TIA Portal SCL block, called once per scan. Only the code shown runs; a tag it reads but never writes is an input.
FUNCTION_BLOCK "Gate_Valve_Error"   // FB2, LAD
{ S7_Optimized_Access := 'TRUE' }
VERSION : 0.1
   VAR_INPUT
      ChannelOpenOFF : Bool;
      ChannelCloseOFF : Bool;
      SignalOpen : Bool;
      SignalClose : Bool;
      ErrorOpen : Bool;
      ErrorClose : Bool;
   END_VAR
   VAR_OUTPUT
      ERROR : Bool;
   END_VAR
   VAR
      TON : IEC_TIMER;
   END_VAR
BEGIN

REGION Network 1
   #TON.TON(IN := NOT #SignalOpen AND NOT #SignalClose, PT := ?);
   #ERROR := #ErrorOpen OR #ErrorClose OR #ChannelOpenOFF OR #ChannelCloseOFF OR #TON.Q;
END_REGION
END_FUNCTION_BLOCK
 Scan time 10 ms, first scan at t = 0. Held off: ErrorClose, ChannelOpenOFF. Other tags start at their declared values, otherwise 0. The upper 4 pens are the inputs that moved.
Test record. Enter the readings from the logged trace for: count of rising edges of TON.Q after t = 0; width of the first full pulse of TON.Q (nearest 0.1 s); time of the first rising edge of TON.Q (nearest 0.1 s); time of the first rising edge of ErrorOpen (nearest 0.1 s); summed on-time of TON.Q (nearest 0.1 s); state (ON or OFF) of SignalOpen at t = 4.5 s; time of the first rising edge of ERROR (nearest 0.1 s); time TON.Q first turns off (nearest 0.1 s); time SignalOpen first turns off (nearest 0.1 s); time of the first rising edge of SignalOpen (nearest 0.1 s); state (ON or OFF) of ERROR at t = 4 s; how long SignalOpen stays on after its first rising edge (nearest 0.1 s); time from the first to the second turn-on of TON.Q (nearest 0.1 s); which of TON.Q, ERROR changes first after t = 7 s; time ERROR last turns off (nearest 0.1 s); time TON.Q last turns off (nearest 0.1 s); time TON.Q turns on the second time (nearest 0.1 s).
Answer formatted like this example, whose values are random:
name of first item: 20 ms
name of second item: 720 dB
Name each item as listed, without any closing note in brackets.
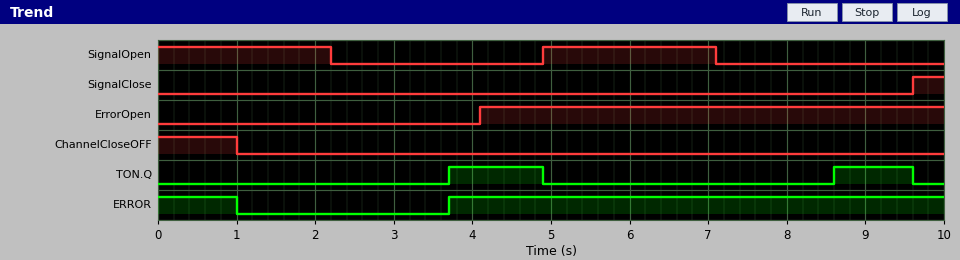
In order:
count of rising edges of TON.Q after t = 0: 2
width of the first full pulse of TON.Q: 1.2 s
time of the first rising edge of TON.Q: 3.7 s
time of the first rising edge of ErrorOpen: 4.1 s
summed on-time of TON.Q: 2.2 s
state (ON or OFF) of SignalOpen at t = 4.5 s: OFF
time of the first rising edge of ERROR: 3.7 s
time TON.Q first turns off: 4.9 s
time SignalOpen first turns off: 2.2 s
time of the first rising edge of SignalOpen: 4.9 s
state (ON or OFF) of ERROR at t = 4 s: ON
how long SignalOpen stays on after its first rising edge: 2.2 s
time from the first to the second turn-on of TON.Q: 4.9 s
which of TON.Q, ERROR changes first after t = 7 s: TON.Q
time ERROR last turns off: 1.0 s
time TON.Q last turns off: 9.6 s
time TON.Q turns on the second time: 8.6 s
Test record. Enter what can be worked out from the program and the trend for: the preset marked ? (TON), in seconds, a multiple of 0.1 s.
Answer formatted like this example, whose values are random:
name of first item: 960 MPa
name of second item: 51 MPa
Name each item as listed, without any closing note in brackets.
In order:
the preset marked ? (TON), in seconds, a multiple of 0.1 s: 1.5 s
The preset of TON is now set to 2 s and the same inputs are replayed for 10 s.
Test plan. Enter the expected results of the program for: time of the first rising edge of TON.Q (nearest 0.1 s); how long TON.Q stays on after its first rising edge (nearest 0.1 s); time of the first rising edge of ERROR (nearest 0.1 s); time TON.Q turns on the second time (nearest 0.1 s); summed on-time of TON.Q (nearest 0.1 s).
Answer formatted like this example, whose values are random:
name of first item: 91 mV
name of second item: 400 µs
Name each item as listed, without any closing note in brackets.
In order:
time of the first rising edge of TON.Q: 4.2 s
how long TON.Q stays on after its first rising edge: 0.7 s
time of the first rising edge of ERROR: 4.1 s
time TON.Q turns on the second time: 9.1 s
summed on-time of TON.Q: 1.2 s
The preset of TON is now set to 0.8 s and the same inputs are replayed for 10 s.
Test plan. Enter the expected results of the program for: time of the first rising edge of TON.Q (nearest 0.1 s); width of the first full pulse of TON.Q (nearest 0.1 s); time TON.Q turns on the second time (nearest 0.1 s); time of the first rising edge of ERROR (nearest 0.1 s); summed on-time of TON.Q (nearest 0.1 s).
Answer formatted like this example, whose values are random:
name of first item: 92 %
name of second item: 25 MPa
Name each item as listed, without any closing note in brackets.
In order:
time of the first rising edge of TON.Q: 3.0 s
width of the first full pulse of TON.Q: 1.9 s
time TON.Q turns on the second time: 7.9 s
time of the first rising edge of ERROR: 3.0 s
summed on-time of TON.Q: 3.6 s
